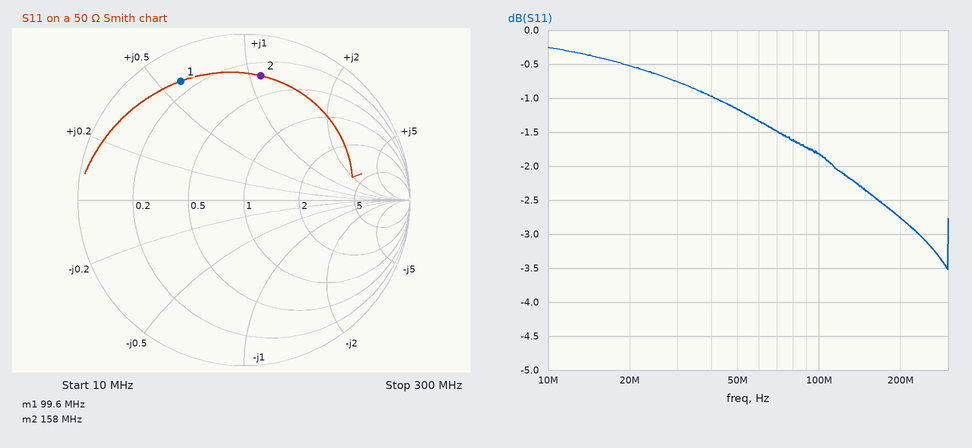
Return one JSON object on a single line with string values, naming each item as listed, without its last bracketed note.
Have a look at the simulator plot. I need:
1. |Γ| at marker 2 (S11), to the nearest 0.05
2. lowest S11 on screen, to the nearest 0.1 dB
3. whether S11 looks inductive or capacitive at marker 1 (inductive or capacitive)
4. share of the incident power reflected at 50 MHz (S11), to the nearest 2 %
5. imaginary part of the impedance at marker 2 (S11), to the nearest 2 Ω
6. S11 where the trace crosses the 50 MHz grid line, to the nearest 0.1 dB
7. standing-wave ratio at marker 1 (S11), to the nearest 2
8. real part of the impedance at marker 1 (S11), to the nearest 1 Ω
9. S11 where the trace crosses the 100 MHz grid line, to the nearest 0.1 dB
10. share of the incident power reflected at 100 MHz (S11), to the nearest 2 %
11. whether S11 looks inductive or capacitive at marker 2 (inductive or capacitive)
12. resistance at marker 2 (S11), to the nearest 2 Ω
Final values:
{"|Γ| at marker 2 (S11), to the nearest 0.05": "0.75", "lowest S11 on screen, to the nearest 0.1 dB": "-3.5 dB", "whether S11 looks inductive or capacitive at marker 1": "inductive", "share of the incident power reflected at 50 MHz (S11), to the nearest 2 %": "76 %", "imaginary part of the impedance at marker 2 (S11), to the nearest 2 Ω": "+54 Ω", "S11 where the trace crosses the 50 MHz grid line, to the nearest 0.1 dB": "-1.2 dB", "standing-wave ratio at marker 1 (S11), to the nearest 2": "10", "real part of the impedance at marker 1 (S11), to the nearest 1 Ω": "7 Ω", "S11 where the trace crosses the 100 MHz grid line, to the nearest 0.1 dB": "-1.8 dB", "share of the incident power reflected at 100 MHz (S11), to the nearest 2 %": "66 %", "whether S11 looks inductive or capacitive at marker 2": "inductive", "resistance at marker 2 (S11), to the nearest 2 Ω": "16 Ω"}
